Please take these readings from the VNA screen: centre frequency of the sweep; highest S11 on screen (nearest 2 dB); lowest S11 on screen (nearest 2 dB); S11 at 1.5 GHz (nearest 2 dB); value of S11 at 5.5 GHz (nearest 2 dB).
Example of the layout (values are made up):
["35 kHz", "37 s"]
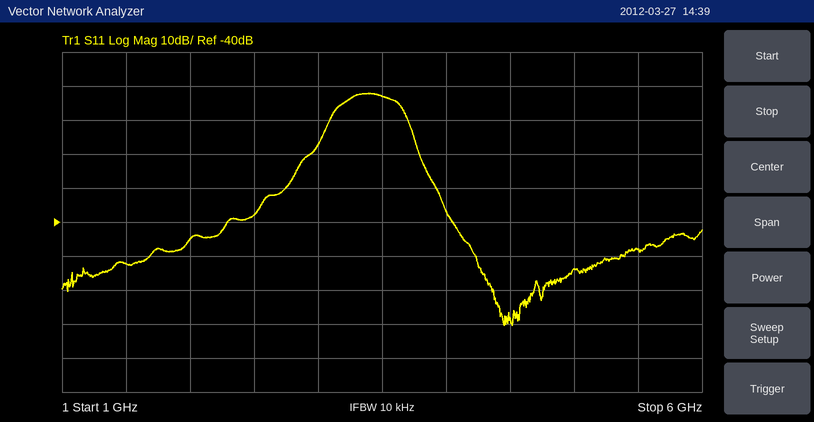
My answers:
["3.5 GHz", "-2 dB", "-70 dB", "-52 dB", "-48 dB"]
